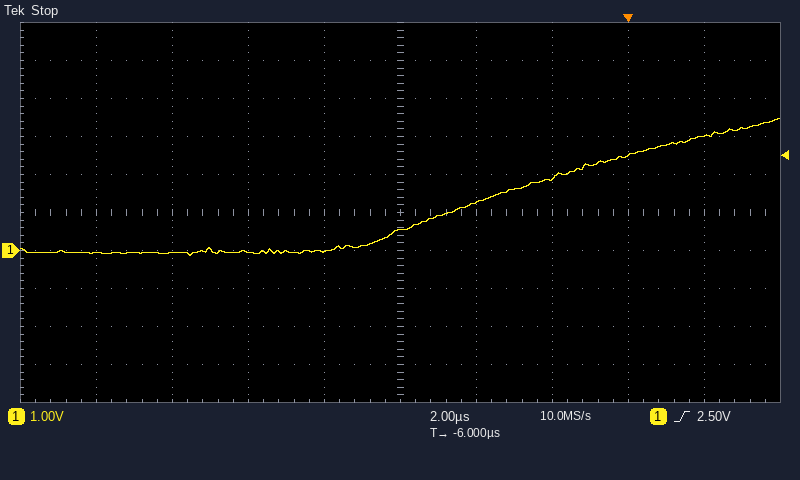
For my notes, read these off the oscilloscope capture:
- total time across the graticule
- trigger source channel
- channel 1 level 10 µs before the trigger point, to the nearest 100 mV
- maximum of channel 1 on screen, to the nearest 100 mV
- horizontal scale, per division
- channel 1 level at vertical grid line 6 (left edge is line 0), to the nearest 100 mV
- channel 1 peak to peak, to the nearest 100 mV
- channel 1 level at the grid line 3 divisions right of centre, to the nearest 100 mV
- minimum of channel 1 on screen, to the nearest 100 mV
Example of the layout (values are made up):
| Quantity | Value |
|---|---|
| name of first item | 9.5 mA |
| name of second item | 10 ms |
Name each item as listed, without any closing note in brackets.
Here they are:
| Quantity | Value |
|---|---|
| total time across the graticule | 20 µs |
| trigger source channel | channel 1 |
| channel 1 level 10 µs before the trigger point, to the nearest 100 mV | 0.0 V |
| maximum of channel 1 on screen, to the nearest 100 mV | 3.5 V |
| horizontal scale, per division | 2 µs |
| channel 1 level at vertical grid line 6 (left edge is line 0), to the nearest 100 mV | 1.3 V |
| channel 1 peak to peak, to the nearest 100 mV | 3.6 V |
| channel 1 level at the grid line 3 divisions right of centre, to the nearest 100 mV | 2.5 V |
| minimum of channel 1 on screen, to the nearest 100 mV | -100 mV |
